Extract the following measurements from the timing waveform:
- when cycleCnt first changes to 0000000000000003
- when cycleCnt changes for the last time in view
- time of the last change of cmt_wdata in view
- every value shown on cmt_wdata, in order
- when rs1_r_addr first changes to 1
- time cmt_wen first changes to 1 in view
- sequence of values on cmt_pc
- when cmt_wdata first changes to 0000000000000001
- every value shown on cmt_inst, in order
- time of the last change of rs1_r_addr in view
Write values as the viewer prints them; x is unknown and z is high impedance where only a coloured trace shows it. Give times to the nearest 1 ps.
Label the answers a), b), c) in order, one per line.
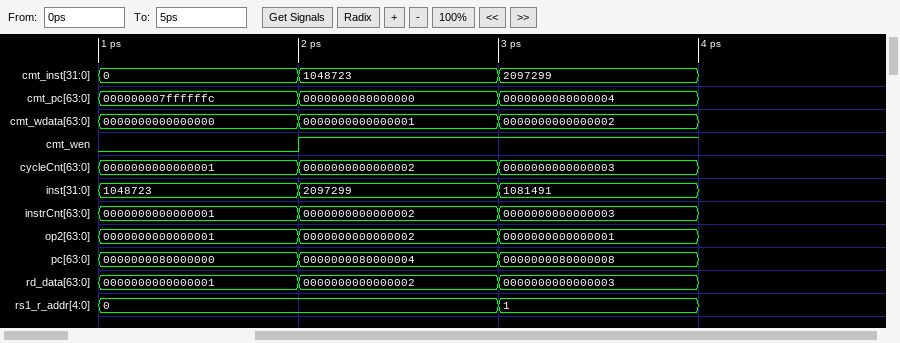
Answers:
a) 3 ps
b) 3 ps
c) 3 ps
d) 0000000000000000, 0000000000000001, 0000000000000002
e) 3 ps
f) 2 ps
g) 000000007ffffffc, 0000000080000000, 0000000080000004
h) 2 ps
i) 0, 1048723, 2097299
j) 3 ps
